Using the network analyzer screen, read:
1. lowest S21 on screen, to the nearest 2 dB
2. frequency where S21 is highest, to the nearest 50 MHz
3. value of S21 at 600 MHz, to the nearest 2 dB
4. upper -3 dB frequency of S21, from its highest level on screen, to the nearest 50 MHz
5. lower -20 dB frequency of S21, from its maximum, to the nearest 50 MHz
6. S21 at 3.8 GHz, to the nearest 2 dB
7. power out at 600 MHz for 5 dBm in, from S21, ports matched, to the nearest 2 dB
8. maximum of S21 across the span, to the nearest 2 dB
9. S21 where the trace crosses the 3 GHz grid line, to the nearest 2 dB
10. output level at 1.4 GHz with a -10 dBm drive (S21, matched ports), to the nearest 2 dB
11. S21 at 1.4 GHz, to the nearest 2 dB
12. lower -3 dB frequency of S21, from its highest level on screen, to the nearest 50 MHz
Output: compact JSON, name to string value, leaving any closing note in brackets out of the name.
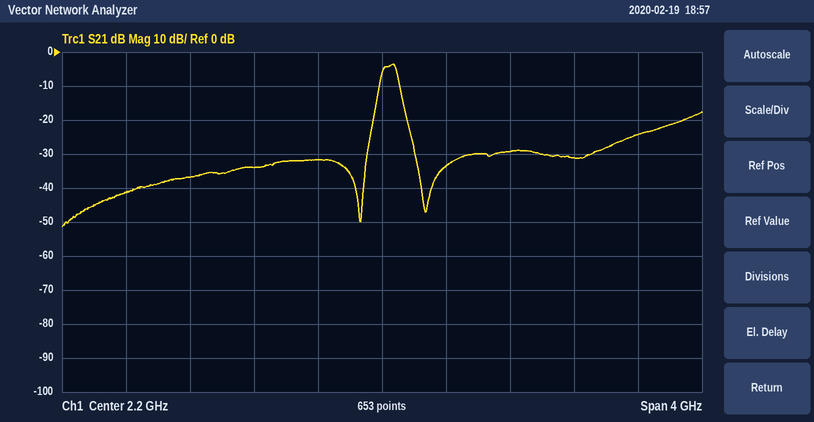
{"lowest S21 on screen, to the nearest 2 dB": "-52 dB", "frequency where S21 is highest, to the nearest 50 MHz": "2.25 GHz", "value of S21 at 600 MHz, to the nearest 2 dB": "-42 dB", "upper -3 dB frequency of S21, from its highest level on screen, to the nearest 50 MHz": "2.30 GHz", "lower -20 dB frequency of S21, from its maximum, to the nearest 50 MHz": "2.15 GHz", "S21 at 3.8 GHz, to the nearest 2 dB": "-24 dB", "power out at 600 MHz for 5 dBm in, from S21, ports matched, to the nearest 2 dB": "-36 dBm", "maximum of S21 across the span, to the nearest 2 dB": "-4 dB", "S21 where the trace crosses the 3 GHz grid line, to the nearest 2 dB": "-30 dB", "output level at 1.4 GHz with a -10 dBm drive (S21, matched ports), to the nearest 2 dB": "-44 dBm", "S21 at 1.4 GHz, to the nearest 2 dB": "-34 dB", "lower -3 dB frequency of S21, from its highest level on screen, to the nearest 50 MHz": "2.20 GHz"}
